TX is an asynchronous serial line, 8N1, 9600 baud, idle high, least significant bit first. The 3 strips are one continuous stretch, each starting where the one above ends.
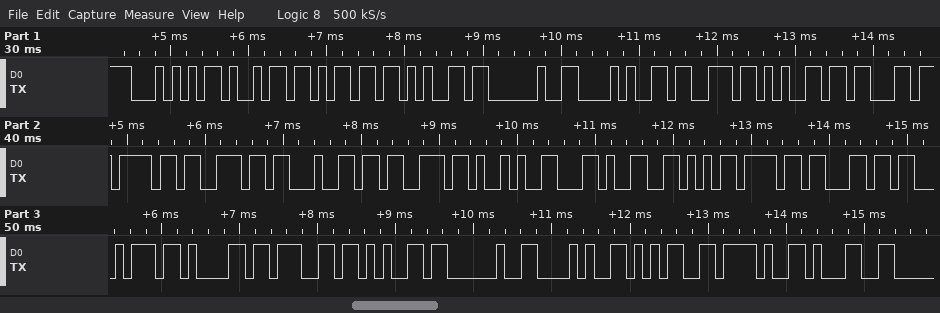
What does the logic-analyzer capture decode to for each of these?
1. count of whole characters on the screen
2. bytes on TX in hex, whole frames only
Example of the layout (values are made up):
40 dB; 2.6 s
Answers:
27; 0x54 0x69 0x6D 0x65 0x20 0x28 0x73 0x65 0x63 0x6F 0x6E 0x64 0x73 0x29 0x2C 0x56 0x6F 0x6C 0x74 0x61 0x67 0x65 0x20 0x28 0x35 0x2F 0x31
